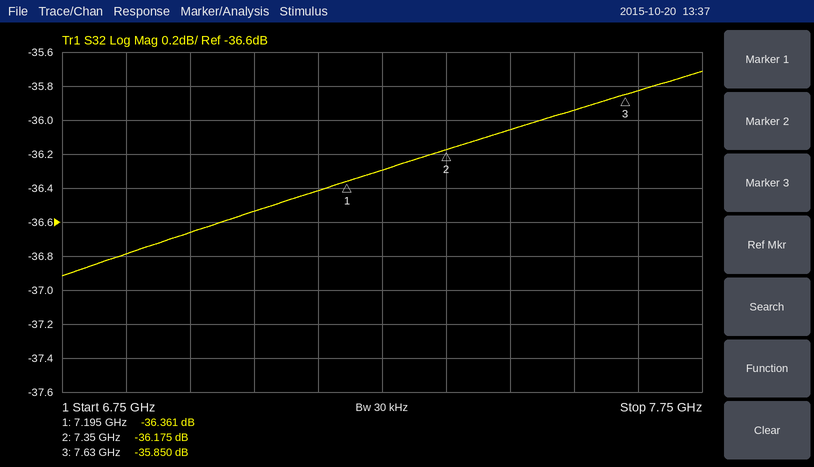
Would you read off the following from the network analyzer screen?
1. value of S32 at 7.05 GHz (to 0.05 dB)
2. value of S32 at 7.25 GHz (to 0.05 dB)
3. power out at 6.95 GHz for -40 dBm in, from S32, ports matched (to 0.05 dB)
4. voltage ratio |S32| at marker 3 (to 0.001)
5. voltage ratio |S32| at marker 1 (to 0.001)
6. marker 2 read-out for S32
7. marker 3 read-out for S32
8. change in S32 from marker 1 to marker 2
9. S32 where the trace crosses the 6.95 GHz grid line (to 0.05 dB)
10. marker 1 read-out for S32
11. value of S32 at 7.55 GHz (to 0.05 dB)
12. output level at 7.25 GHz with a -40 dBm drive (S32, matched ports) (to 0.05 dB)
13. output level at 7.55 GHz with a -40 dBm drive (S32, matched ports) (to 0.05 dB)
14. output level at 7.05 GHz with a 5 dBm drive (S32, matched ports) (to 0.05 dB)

-36.55 dB
-36.30 dB
-76.65 dBm
0.016
0.015
-36.175 dB
-35.850 dB
0.186 dB
-36.65 dB
-36.361 dB
-35.95 dB
-76.30 dBm
-75.95 dBm
-31.55 dBm
